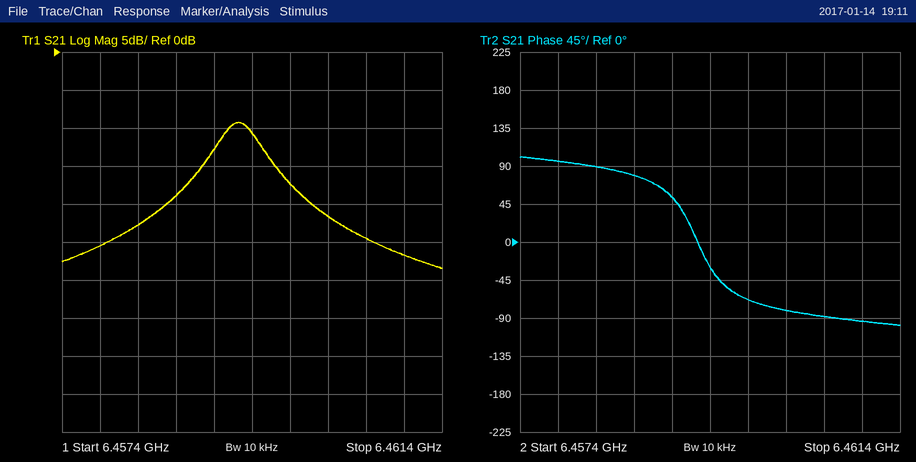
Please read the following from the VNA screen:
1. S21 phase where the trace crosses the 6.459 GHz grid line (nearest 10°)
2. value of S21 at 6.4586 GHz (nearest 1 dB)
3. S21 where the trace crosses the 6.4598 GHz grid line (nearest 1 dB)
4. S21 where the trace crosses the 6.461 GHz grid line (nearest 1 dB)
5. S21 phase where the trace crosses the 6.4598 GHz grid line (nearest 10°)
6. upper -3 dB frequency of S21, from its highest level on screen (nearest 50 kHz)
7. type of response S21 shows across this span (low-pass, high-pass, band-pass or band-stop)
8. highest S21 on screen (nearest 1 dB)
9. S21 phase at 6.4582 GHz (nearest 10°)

50°
-19 dB
-17 dB
-27 dB
-70°
6.45950 GHz
band-pass
-9 dB
90°
